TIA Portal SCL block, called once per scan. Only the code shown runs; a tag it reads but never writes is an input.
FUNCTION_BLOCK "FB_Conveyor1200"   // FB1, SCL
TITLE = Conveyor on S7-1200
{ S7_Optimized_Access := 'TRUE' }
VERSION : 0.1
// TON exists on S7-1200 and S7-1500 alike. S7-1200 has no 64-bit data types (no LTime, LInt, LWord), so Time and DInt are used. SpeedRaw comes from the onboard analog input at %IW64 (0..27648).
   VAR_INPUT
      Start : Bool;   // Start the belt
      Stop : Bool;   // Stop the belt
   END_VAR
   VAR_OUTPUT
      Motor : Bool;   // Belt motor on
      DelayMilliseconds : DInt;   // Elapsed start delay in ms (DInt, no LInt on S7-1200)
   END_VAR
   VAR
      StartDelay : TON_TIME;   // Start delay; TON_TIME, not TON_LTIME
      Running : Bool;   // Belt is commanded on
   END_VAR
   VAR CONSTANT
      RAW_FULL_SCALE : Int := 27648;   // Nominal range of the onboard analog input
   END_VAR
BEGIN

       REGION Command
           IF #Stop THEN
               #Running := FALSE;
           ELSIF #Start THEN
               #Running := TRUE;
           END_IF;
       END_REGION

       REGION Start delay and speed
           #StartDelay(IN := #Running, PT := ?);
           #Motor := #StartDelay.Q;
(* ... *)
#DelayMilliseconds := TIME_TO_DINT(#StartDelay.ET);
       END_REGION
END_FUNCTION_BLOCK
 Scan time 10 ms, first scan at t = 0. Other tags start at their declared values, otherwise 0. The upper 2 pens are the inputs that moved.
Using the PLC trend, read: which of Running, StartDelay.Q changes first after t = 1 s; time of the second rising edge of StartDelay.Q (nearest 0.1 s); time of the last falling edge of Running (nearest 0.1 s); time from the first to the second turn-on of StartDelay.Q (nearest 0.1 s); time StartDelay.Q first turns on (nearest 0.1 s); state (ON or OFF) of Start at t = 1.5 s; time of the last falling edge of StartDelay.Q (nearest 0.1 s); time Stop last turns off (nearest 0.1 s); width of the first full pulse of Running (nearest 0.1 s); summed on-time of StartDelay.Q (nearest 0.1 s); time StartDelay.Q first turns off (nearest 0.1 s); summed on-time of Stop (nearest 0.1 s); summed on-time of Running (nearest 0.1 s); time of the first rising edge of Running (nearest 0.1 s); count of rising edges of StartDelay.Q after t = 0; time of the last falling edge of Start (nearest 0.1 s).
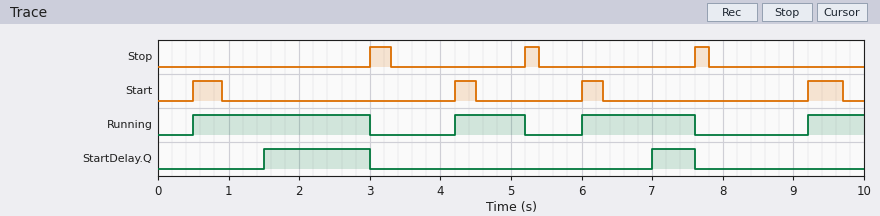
StartDelay.Q
7.0 s
7.6 s
5.5 s
1.5 s
OFF
7.6 s
7.8 s
2.5 s
2.1 s
3.0 s
0.7 s
5.9 s
0.5 s
2
9.7 s
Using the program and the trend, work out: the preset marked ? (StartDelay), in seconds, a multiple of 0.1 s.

1.0 s
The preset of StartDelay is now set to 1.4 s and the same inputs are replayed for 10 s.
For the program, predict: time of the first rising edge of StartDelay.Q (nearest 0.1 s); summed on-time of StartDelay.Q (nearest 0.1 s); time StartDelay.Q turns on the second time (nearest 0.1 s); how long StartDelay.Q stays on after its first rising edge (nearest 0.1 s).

1.9 s
1.3 s
7.4 s
1.1 s
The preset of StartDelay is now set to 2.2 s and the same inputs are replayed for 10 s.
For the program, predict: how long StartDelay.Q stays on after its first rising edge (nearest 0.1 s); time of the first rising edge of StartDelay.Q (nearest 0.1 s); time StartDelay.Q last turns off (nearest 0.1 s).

0.3 s
2.7 s
3.0 s
